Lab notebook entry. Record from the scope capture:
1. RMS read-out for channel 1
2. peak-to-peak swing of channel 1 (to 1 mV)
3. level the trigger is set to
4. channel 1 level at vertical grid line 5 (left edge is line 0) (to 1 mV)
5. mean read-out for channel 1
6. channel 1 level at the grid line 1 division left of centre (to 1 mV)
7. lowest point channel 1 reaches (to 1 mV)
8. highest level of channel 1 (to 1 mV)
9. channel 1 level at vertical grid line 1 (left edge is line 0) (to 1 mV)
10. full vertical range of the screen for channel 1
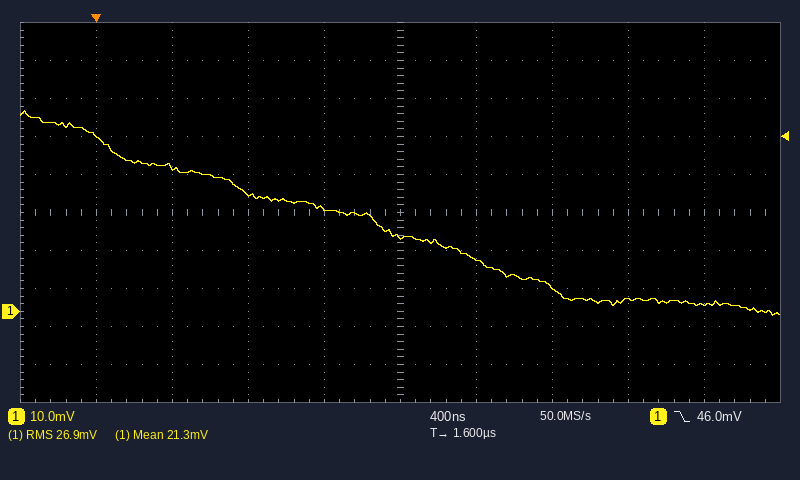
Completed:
26.9 mV
54 mV
46.0 mV
20 mV
21.3 mV
27 mV
-1 mV
53 mV
46 mV
100 mV
